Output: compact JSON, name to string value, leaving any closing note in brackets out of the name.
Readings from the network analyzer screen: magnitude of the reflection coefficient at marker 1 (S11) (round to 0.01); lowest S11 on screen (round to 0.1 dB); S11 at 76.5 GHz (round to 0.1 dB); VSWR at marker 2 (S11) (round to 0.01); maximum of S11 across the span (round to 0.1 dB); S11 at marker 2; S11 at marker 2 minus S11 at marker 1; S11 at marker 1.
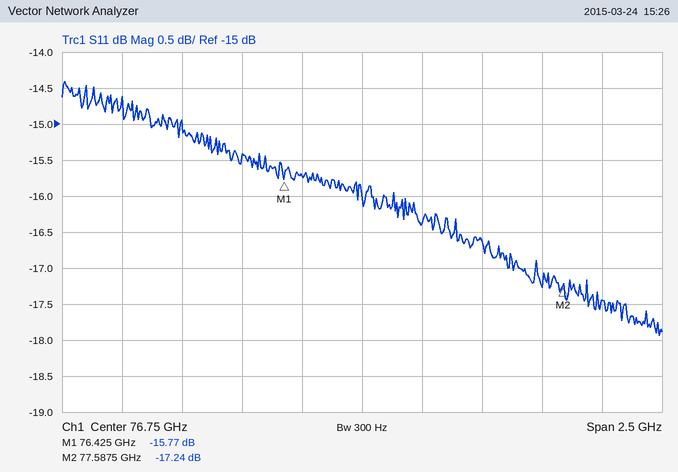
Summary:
{"magnitude of the reflection coefficient at marker 1 (S11)": "0.16", "lowest S11 on screen": "-17.9 dB", "S11 at 76.5 GHz": "-15.7 dB", "VSWR at marker 2 (S11)": "1.32", "maximum of S11 across the span": "-14.4 dB", "S11 at marker 2": "-17.24 dB", "S11 at marker 2 minus S11 at marker 1": "-1.47 dB", "S11 at marker 1": "-15.77 dB"}
